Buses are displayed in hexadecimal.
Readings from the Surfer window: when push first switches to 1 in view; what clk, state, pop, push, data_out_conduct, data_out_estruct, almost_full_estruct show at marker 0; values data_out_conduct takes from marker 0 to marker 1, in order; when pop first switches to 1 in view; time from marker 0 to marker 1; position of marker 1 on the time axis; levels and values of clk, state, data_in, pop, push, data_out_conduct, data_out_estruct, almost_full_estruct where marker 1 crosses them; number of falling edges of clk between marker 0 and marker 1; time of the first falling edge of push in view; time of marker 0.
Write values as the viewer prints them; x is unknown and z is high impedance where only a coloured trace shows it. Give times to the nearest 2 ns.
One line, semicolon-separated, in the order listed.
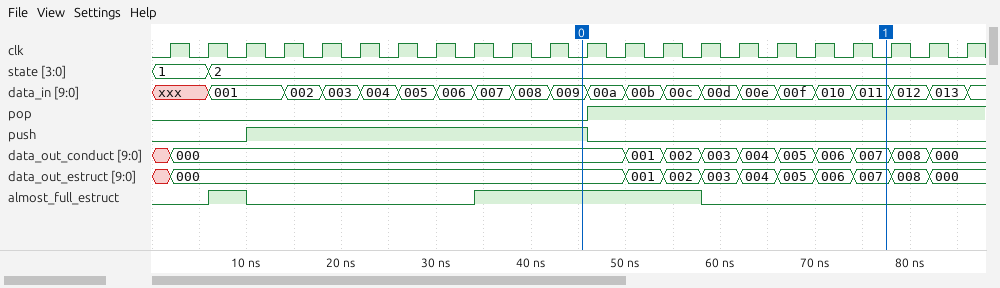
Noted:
10 ns; clk=0, state=2, pop=0, push=1, data_out_conduct=000, data_out_estruct=000, almost_full_estruct=1; 000, 001, 002, 003, 004, 005, 006, 007; 46 ns; 32 ns; 78 ns; clk=0, state=2, data_in=011, pop=1, push=0, data_out_conduct=007, data_out_estruct=007, almost_full_estruct=0; 8; 46 ns; 46 ns
